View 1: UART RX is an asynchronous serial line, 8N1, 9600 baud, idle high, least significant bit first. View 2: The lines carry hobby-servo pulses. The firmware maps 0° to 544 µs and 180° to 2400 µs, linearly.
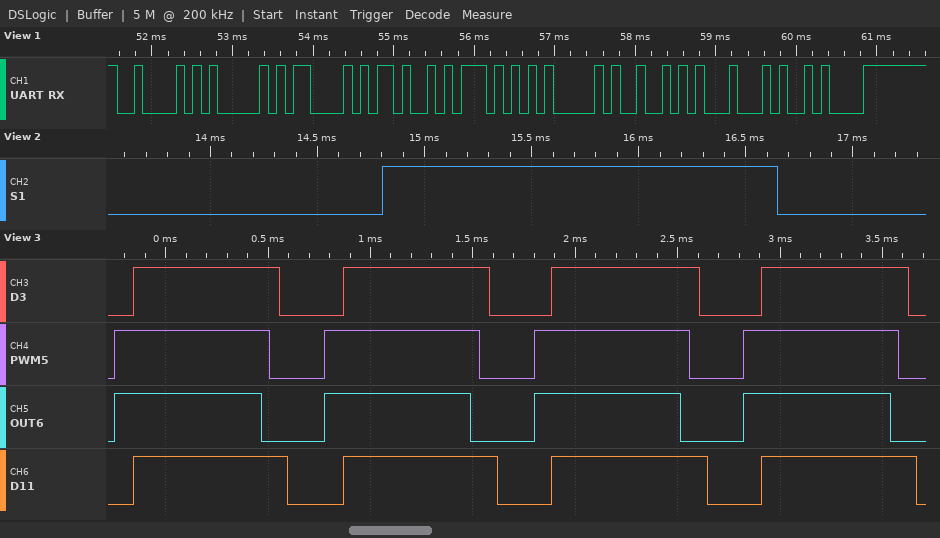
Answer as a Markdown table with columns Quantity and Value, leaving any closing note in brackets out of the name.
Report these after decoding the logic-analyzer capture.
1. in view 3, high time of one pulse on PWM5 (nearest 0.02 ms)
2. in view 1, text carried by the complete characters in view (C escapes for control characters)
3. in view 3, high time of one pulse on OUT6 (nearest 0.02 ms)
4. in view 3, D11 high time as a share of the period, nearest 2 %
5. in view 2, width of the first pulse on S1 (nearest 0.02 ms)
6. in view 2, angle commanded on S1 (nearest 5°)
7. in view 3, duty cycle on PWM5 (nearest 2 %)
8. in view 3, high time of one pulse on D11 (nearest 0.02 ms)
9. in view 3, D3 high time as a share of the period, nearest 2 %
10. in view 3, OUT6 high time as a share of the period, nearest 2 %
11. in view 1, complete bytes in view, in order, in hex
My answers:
| Quantity | Value |
|---|---|
| in view 3, high time of one pulse on PWM5 | 0.76 ms |
| in view 1, text carried by the complete characters in view | "BACKWARD\n" |
| in view 3, high time of one pulse on OUT6 | 0.72 ms |
| in view 3, D11 high time as a share of the period, nearest 2 % | 74 % |
| in view 2, width of the first pulse on S1 | 1.84 ms |
| in view 2, angle commanded on S1 | 125° |
| in view 3, duty cycle on PWM5 | 74 % |
| in view 3, high time of one pulse on D11 | 0.76 ms |
| in view 3, D3 high time as a share of the period, nearest 2 % | 70 % |
| in view 3, OUT6 high time as a share of the period, nearest 2 % | 70 % |
| in view 1, complete bytes in view, in order, in hex | 42 41 43 4B 57 41 52 44 0A |
